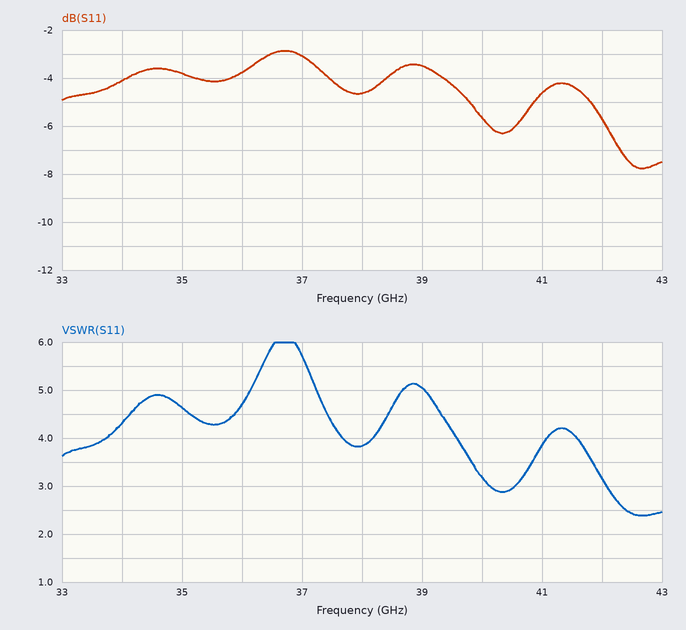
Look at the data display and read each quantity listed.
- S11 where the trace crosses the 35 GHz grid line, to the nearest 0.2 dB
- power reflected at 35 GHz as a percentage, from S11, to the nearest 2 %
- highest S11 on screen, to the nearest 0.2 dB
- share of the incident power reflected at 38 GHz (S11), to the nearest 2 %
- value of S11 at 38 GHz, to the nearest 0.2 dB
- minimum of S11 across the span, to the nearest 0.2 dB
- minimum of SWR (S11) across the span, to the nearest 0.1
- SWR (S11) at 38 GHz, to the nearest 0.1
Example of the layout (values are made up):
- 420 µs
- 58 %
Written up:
- -3.8 dB
- 42 %
- -2.8 dB
- 34 %
- -4.6 dB
- -7.8 dB
- 2.4
- 3.8
